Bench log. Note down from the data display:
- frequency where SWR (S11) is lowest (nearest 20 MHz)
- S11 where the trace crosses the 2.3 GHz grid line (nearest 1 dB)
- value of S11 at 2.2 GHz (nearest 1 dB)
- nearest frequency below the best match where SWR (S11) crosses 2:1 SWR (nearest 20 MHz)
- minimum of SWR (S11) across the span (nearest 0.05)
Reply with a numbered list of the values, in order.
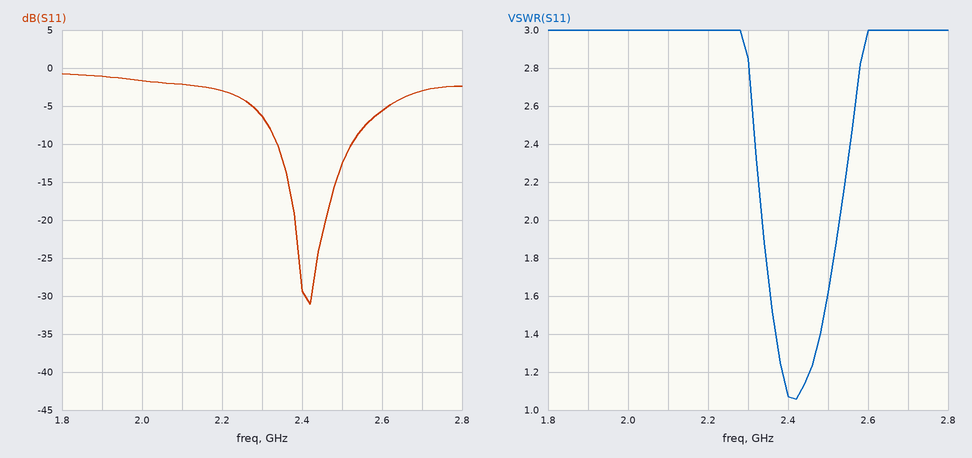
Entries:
1. 2.42 GHz
2. -6 dB
3. -3 dB
4. 2.34 GHz
5. 1.05
